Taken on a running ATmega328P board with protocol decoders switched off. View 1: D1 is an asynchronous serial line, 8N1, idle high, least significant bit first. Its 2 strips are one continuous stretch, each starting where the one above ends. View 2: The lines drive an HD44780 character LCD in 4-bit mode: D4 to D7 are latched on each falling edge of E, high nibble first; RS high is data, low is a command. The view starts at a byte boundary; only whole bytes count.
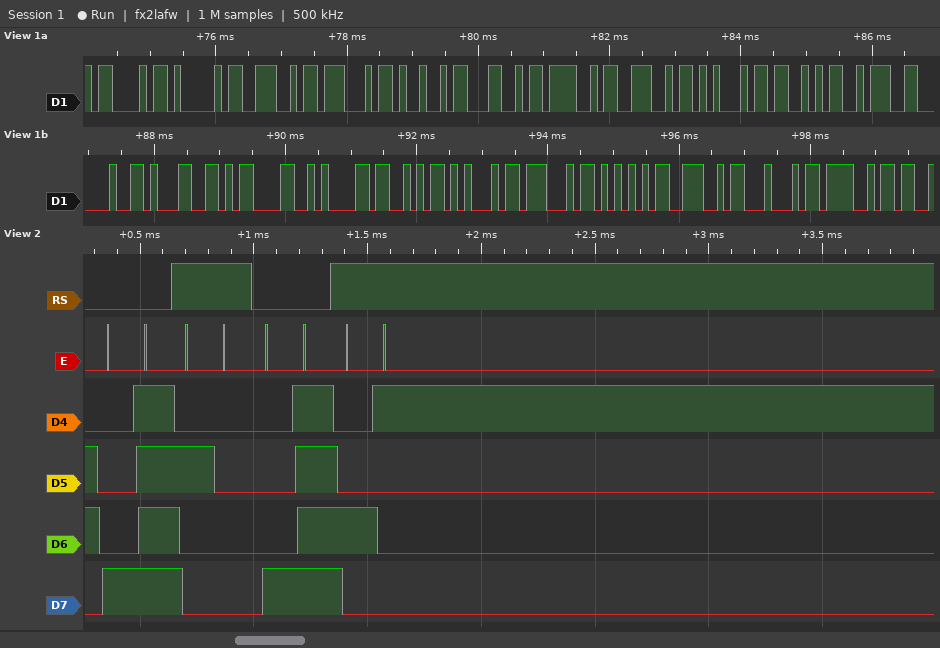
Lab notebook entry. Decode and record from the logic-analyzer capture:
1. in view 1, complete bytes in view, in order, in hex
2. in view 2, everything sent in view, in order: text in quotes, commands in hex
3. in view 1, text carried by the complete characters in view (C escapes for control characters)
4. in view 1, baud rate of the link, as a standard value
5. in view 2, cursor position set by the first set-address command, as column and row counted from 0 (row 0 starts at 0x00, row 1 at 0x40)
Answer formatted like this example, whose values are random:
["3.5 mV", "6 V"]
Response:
["43 41 4E 47 49 4C 4F 4E 45 53 3A 20 31 0D 0A 53 45 47 55 4E 44 4F", "0x8F \" \" 0x8F \"A\"", "\"CANGILONES: 1\\r\\nSEGUNDO\"", "9600 baud", "column 15, row 0"]
